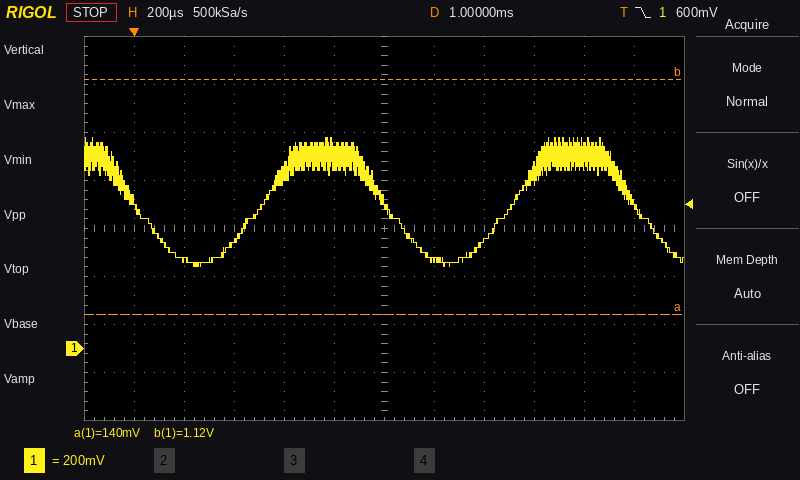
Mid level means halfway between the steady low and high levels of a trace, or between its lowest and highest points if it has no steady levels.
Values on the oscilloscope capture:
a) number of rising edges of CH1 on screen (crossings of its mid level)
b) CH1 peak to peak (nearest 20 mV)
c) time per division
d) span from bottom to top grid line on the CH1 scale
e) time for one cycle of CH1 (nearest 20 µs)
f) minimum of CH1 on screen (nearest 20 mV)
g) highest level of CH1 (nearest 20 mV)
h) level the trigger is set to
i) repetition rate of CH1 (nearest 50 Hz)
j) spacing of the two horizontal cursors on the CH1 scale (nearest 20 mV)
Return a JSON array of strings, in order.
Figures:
["2", "540 mV", "200 µs", "1.6 V", "1.00 ms", "340 mV", "880 mV", "600 mV", "1.00 kHz", "980 mV"]
